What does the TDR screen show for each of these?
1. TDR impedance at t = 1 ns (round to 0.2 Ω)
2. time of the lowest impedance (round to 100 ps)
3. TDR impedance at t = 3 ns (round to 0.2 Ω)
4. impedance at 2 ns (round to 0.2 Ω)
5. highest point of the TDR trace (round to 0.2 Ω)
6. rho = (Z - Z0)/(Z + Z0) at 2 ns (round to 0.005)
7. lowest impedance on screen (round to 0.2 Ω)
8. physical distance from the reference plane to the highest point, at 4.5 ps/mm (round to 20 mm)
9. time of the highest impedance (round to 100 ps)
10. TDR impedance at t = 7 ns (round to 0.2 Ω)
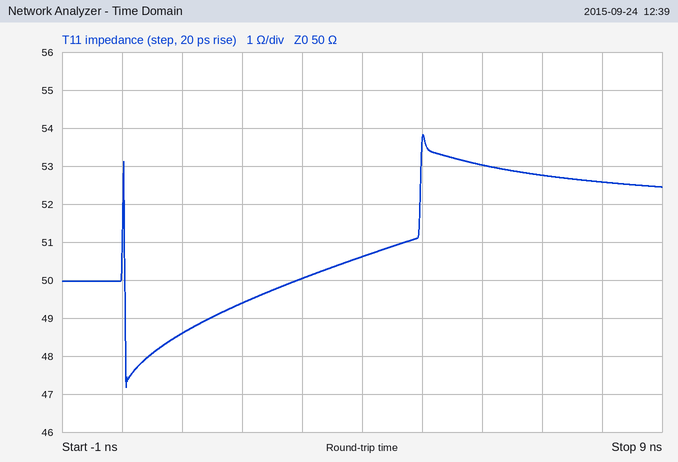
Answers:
48.6 Ω
100 ps
50.0 Ω
49.4 Ω
53.8 Ω
-0.005
47.2 Ω
560 mm
5.0 ns
52.8 Ω
